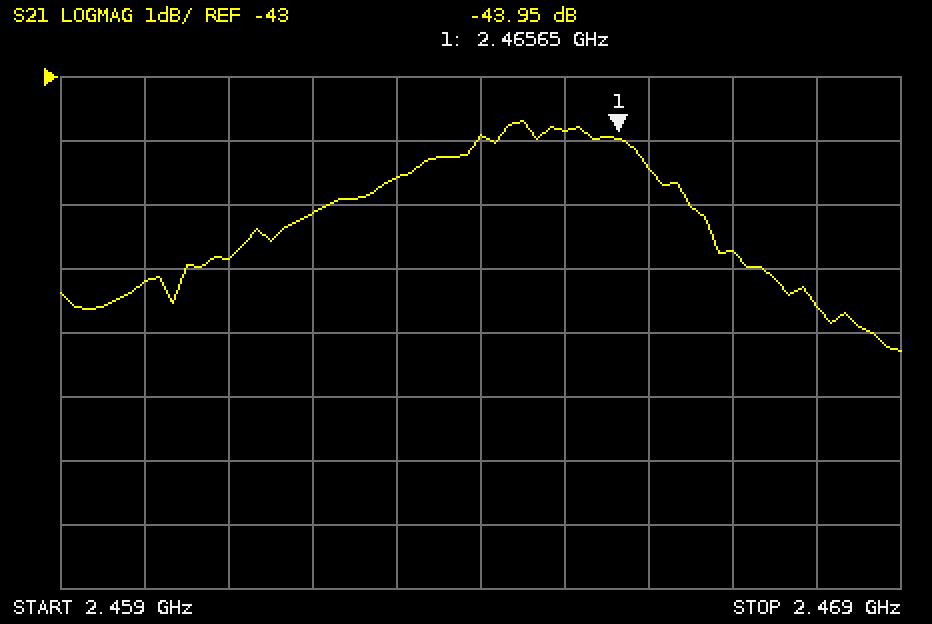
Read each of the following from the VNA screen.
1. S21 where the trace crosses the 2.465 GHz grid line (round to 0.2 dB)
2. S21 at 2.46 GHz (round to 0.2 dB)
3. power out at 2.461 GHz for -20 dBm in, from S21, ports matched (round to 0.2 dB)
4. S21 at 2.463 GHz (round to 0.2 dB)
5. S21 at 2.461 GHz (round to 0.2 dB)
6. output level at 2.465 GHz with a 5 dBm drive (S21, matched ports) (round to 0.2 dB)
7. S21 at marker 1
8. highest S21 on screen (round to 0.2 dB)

-43.8 dB
-46.2 dB
-65.8 dBm
-44.6 dB
-45.8 dB
-38.8 dBm
-43.95 dB
-43.6 dB
